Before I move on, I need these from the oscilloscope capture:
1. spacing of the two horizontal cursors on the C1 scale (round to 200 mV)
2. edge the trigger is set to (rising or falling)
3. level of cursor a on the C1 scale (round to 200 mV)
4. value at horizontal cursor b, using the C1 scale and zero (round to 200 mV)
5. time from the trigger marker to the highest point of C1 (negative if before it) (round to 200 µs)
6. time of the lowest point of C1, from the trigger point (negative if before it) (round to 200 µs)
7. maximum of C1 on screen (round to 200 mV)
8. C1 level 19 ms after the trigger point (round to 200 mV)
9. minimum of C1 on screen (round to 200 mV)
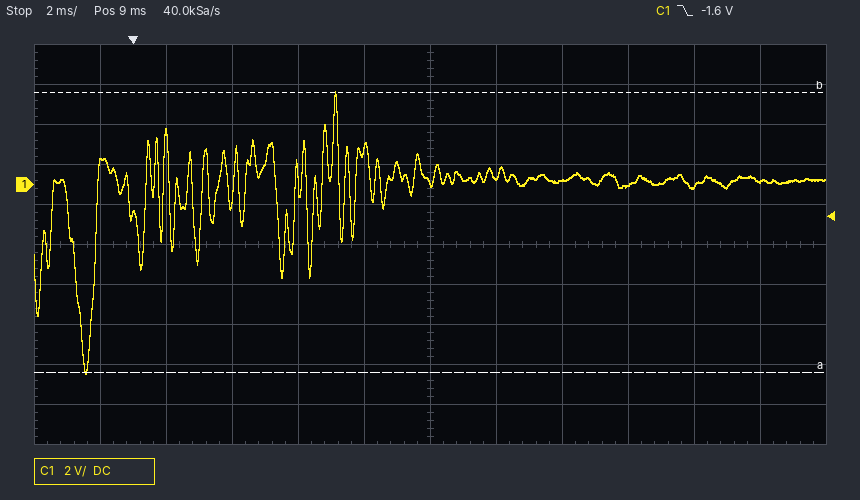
14.0 V
falling
-9.4 V
4.6 V
+6.2 ms
-1.4 ms
4.6 V
200 mV
-9.4 V
